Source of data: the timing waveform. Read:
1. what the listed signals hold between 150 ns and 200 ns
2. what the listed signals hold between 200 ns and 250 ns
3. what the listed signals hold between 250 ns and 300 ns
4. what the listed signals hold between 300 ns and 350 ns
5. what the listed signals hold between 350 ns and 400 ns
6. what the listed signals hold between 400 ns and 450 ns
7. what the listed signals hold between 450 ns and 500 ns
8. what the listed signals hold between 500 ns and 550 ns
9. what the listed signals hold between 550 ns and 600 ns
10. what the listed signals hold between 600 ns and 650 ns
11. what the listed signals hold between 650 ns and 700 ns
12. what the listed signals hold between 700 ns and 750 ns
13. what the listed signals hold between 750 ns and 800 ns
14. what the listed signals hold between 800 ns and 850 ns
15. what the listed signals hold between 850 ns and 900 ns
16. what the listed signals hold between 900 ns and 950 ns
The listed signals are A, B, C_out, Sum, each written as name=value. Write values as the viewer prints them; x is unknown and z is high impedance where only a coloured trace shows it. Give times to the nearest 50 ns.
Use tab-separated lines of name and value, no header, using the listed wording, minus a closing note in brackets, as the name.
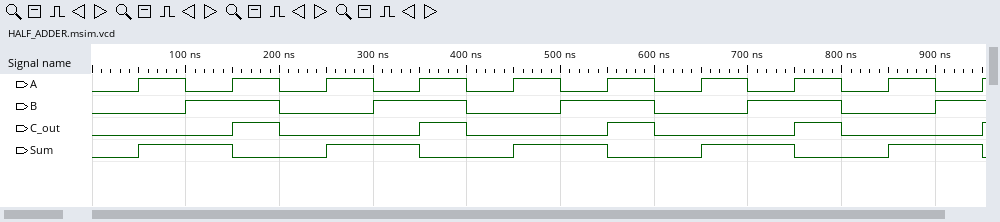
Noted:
what the listed signals hold between 150 ns and 200 ns	A=1, B=1, C_out=1, Sum=0
what the listed signals hold between 200 ns and 250 ns	A=0, B=0, C_out=0, Sum=0
what the listed signals hold between 250 ns and 300 ns	A=1, B=0, C_out=0, Sum=1
what the listed signals hold between 300 ns and 350 ns	A=0, B=1, C_out=0, Sum=1
what the listed signals hold between 350 ns and 400 ns	A=1, B=1, C_out=1, Sum=0
what the listed signals hold between 400 ns and 450 ns	A=0, B=0, C_out=0, Sum=0
what the listed signals hold between 450 ns and 500 ns	A=1, B=0, C_out=0, Sum=1
what the listed signals hold between 500 ns and 550 ns	A=0, B=1, C_out=0, Sum=1
what the listed signals hold between 550 ns and 600 ns	A=1, B=1, C_out=1, Sum=0
what the listed signals hold between 600 ns and 650 ns	A=0, B=0, C_out=0, Sum=0
what the listed signals hold between 650 ns and 700 ns	A=1, B=0, C_out=0, Sum=1
what the listed signals hold between 700 ns and 750 ns	A=0, B=1, C_out=0, Sum=1
what the listed signals hold between 750 ns and 800 ns	A=1, B=1, C_out=1, Sum=0
what the listed signals hold between 800 ns and 850 ns	A=0, B=0, C_out=0, Sum=0
what the listed signals hold between 850 ns and 900 ns	A=1, B=0, C_out=0, Sum=1
what the listed signals hold between 900 ns and 950 ns	A=0, B=1, C_out=0, Sum=1
